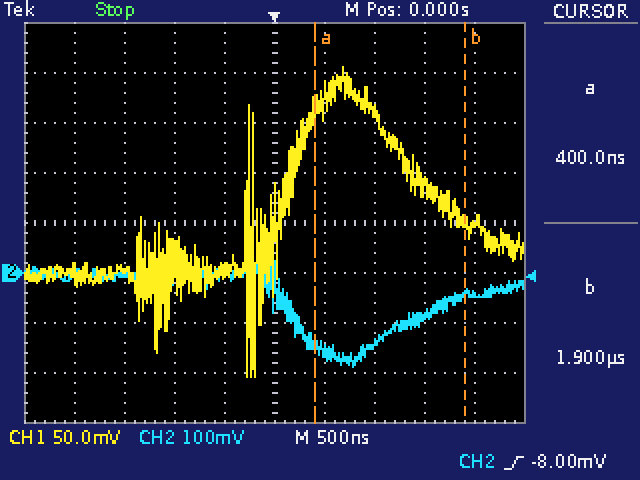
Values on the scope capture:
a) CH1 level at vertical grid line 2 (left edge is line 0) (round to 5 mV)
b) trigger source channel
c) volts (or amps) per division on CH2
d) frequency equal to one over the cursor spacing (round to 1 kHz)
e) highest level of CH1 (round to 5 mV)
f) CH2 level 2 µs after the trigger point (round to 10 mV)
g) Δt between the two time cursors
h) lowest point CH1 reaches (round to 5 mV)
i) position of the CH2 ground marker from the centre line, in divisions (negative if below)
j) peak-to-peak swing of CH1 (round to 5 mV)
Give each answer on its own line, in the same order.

5 mV
CH2
100 mV
667 kHz
205 mV
-40 mV
1.50 µs
-105 mV
-1.0 div
310 mV
